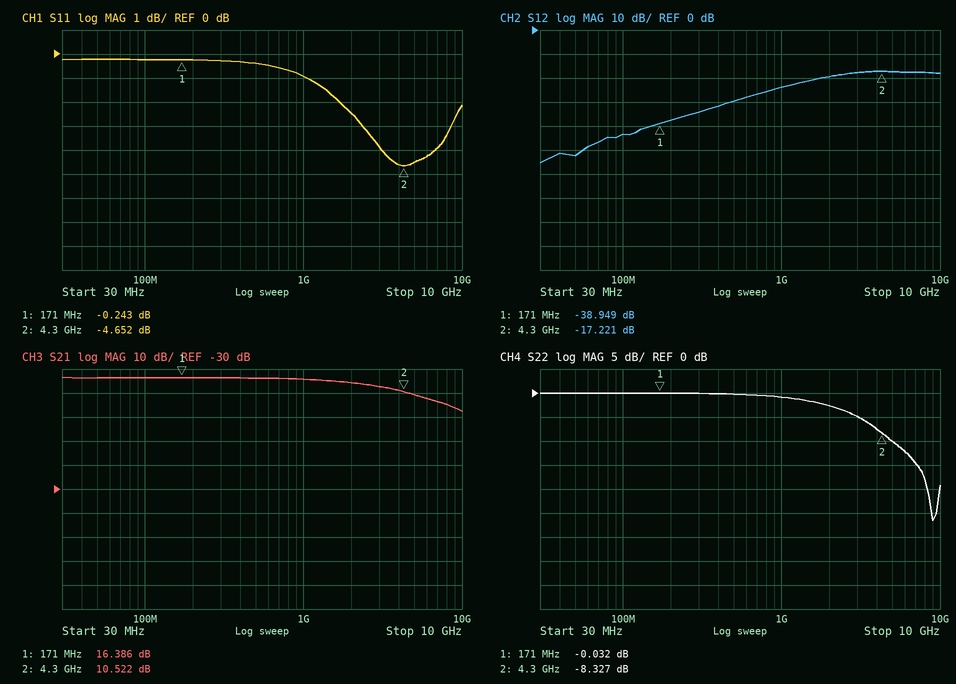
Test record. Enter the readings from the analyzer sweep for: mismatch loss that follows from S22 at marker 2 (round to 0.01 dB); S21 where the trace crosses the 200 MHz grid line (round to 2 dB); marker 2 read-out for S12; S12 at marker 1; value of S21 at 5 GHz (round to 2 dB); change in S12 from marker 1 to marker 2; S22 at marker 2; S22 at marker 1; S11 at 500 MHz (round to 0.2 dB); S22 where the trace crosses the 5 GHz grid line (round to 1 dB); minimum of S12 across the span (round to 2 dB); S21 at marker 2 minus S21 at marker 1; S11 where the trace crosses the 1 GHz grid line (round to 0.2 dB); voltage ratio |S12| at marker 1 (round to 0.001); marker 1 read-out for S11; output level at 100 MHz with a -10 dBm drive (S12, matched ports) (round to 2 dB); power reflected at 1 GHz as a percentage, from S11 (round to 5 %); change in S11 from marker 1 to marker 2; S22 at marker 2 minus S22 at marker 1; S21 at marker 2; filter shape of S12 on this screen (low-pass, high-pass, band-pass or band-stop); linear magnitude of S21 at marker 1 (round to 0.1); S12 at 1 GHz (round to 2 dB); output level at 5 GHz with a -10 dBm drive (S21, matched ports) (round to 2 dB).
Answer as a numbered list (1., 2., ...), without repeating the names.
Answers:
1. 0.69 dB
2. 16 dB
3. -17.221 dB
4. -38.949 dB
5. 10 dB
6. 21.728 dB
7. -8.327 dB
8. -0.032 dB
9. -0.4 dB
10. -10 dB
11. -56 dB
12. -5.864 dB
13. -1.0 dB
14. 0.011
15. -0.243 dB
16. -54 dBm
17. 80 %
18. -4.409 dB
19. -8.295 dB
20. 10.522 dB
21. high-pass
22. 6.6
23. -24 dB
24. 0 dBm
